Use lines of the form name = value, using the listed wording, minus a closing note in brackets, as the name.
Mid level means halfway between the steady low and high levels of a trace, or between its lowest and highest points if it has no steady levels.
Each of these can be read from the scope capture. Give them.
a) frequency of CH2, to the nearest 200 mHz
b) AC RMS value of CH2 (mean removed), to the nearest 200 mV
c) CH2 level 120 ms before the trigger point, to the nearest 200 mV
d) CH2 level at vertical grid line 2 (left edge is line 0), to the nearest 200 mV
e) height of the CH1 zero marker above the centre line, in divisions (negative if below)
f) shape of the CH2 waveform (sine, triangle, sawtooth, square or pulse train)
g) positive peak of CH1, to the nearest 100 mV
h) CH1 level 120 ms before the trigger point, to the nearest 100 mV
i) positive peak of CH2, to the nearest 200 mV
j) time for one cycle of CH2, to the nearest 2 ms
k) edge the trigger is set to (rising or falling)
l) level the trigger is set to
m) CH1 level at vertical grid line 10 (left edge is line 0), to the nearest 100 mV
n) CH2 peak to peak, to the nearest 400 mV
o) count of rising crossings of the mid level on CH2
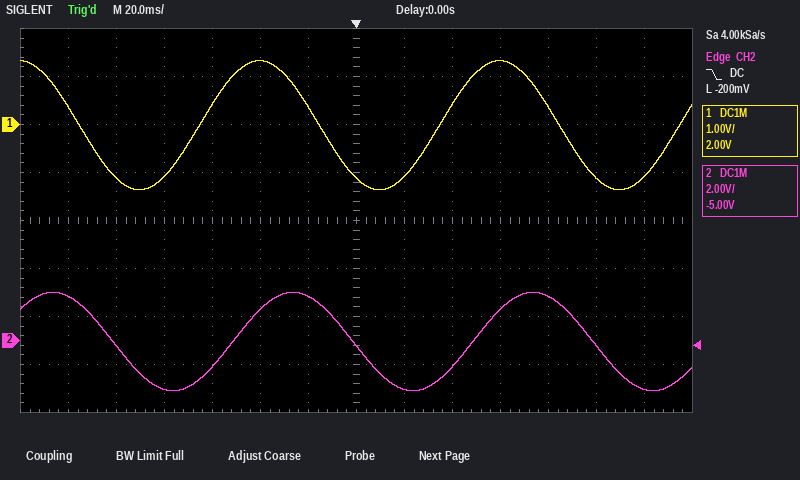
frequency of CH2, to the nearest 200 mHz = 10.0 Hz
AC RMS value of CH2 (mean removed), to the nearest 200 mV = 1.4 V
CH2 level 120 ms before the trigger point, to the nearest 200 mV = 1.8 V
CH2 level at vertical grid line 2 (left edge is line 0), to the nearest 200 mV = -200 mV
height of the CH1 zero marker above the centre line, in divisions = +2.0 div
shape of the CH2 waveform = sine
positive peak of CH1, to the nearest 100 mV = 1.3 V
CH1 level 120 ms before the trigger point, to the nearest 100 mV = 400 mV
positive peak of CH2, to the nearest 200 mV = 2.0 V
time for one cycle of CH2, to the nearest 2 ms = 100 ms
edge the trigger is set to = falling
level the trigger is set to = -200 mV
CH1 level at vertical grid line 10 (left edge is line 0), to the nearest 100 mV = 1.3 V
CH2 peak to peak, to the nearest 400 mV = 4.0 V
count of rising crossings of the mid level on CH2 = 2
